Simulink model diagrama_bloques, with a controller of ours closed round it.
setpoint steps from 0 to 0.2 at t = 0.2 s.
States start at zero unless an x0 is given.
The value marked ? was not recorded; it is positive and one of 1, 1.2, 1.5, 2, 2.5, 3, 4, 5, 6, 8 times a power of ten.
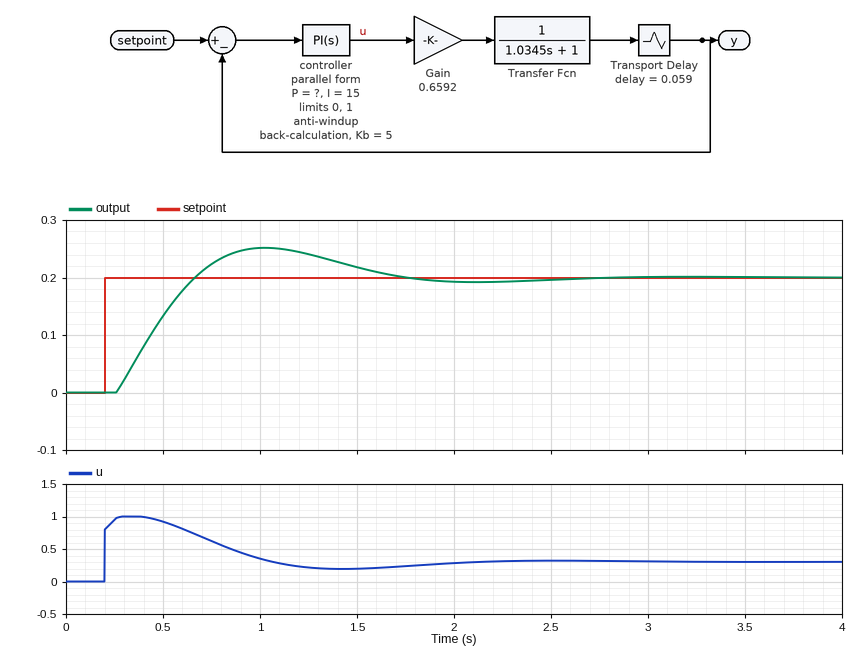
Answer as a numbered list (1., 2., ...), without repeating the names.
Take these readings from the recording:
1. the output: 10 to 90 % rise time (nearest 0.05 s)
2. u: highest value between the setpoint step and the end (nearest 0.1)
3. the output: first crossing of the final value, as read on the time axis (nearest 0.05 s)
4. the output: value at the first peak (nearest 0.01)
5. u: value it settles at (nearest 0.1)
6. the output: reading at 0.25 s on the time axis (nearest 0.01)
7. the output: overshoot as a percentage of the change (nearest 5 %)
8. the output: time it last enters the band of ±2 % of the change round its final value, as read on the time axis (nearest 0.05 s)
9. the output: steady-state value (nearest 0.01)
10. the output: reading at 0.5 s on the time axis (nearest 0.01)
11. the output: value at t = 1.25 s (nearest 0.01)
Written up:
1. 0.30 s
2. 1.0
3. 0.65 s
4. 0.25
5. 0.3
6. 0.00
7. 25 %
8. 2.50 s
9. 0.20
10. 0.13
11. 0.24
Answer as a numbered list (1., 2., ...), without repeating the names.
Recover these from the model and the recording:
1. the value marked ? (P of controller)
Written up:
1. 4
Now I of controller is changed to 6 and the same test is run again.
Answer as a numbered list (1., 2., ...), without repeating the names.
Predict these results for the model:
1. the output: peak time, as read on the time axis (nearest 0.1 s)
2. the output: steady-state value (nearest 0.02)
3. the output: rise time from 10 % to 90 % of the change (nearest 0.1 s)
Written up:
1. 1.5 s
2. 0.20
3. 0.5 s
